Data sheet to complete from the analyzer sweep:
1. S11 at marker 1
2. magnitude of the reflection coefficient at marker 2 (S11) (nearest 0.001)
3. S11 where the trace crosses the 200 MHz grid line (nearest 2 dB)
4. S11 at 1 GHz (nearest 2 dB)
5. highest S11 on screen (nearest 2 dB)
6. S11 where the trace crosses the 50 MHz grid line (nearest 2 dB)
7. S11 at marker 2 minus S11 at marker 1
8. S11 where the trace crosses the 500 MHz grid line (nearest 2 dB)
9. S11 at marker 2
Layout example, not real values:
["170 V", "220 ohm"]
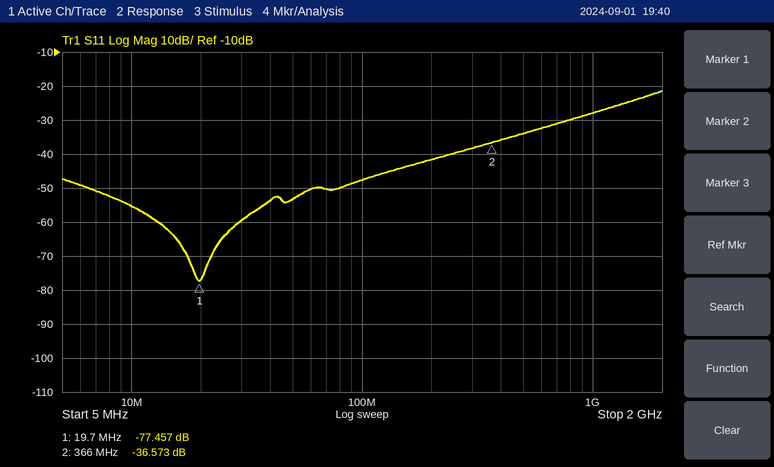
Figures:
["-77.457 dB", "0.015", "-42 dB", "-28 dB", "-22 dB", "-54 dB", "40.884 dB", "-34 dB", "-36.573 dB"]
